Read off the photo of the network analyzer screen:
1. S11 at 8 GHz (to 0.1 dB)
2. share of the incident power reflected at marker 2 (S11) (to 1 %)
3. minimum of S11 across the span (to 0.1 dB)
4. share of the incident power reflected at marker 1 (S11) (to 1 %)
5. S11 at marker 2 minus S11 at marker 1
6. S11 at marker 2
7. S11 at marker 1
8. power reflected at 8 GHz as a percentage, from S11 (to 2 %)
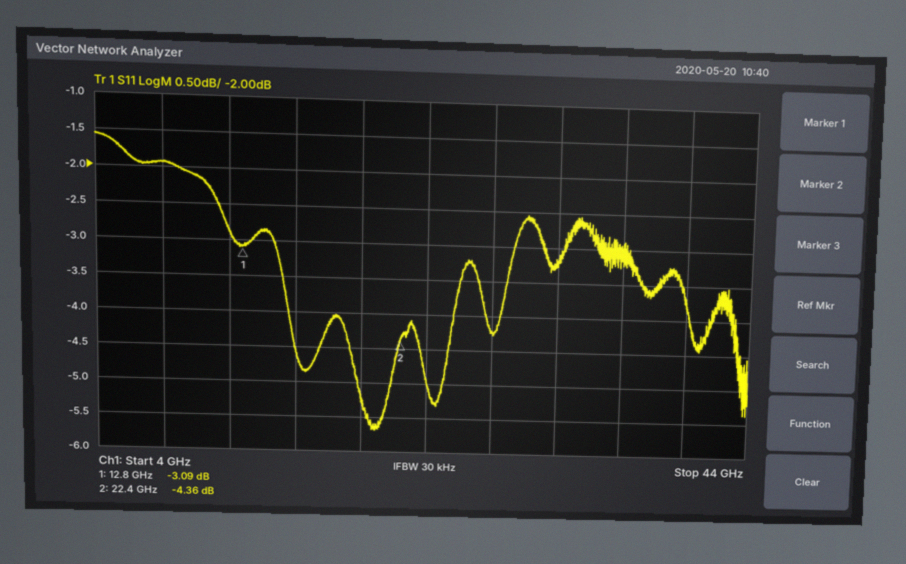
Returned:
-1.9 dB
37 %
-5.7 dB
49 %
-1.27 dB
-4.36 dB
-3.09 dB
64 %
